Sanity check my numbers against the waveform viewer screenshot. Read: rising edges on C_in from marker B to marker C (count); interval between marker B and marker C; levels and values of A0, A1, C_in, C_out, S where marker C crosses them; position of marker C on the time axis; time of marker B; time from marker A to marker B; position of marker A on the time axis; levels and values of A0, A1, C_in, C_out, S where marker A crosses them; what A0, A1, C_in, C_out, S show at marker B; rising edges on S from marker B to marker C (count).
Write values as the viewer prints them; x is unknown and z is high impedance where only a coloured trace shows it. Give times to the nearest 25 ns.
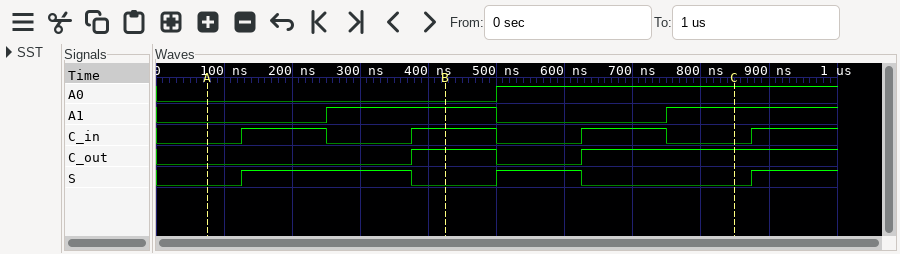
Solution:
1
425 ns
A0=1, A1=1, C_in=0, C_out=1, S=0
850 ns
425 ns
350 ns
75 ns
A0=0, A1=0, C_in=0, C_out=0, S=0
A0=0, A1=1, C_in=1, C_out=1, S=0
1
